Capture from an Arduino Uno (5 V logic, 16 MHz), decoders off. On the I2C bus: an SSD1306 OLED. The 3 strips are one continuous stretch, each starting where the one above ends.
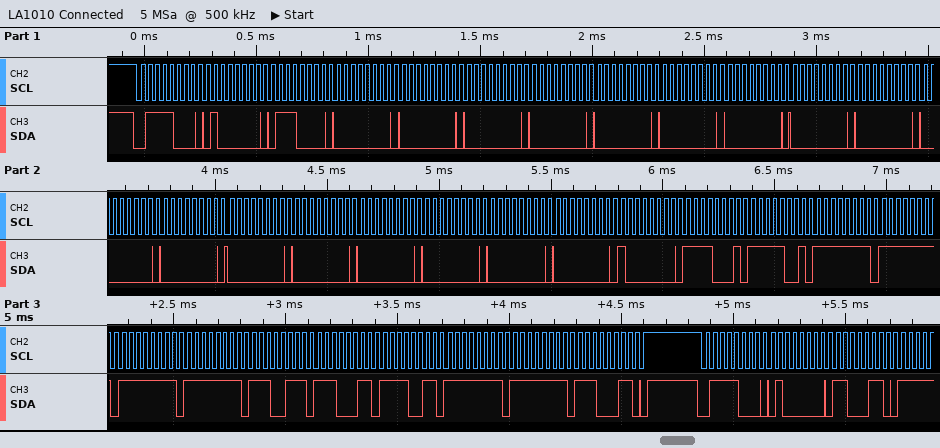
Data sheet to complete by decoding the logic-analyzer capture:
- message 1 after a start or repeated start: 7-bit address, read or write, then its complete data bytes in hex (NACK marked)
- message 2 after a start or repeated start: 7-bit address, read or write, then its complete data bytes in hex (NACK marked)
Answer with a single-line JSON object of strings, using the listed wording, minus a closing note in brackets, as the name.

{"message 1 after a start or repeated start: 7-bit address, read or write, then its complete data bytes in hex": "0x3C write: 40 70 00 00 00 00 00 00 00 00 00 00 00 00 00 00 00 00 00 80 F1 F9 FF FF FF FF E7 E3 F3 FF FF E3", "message 2 after a start or repeated start: 7-bit address, read or write, then its complete data bytes in hex": "0x3C write: 40 C6"}
